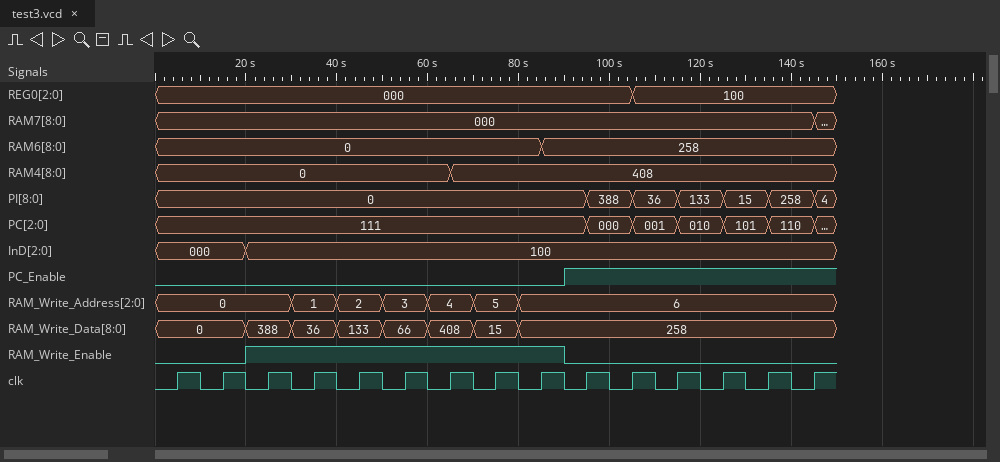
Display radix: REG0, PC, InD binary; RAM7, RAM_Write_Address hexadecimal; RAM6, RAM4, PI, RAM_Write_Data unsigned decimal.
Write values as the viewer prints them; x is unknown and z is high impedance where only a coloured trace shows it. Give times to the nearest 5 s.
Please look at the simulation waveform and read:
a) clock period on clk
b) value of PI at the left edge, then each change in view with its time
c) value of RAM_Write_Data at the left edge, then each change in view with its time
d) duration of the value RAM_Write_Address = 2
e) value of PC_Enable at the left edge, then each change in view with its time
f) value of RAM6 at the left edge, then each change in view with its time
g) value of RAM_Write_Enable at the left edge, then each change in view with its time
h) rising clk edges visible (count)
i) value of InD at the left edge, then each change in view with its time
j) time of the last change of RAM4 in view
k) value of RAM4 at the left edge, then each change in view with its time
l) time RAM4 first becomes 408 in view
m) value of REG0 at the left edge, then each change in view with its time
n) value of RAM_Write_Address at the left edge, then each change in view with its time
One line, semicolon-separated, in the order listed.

10 s; 0, 388 at 95 s, 36 at 105 s, 133 at 115 s, 15 at 125 s, 258 at 135 s, 4 at 145 s; 0, 388 at 20 s, 36 at 30 s, 133 at 40 s, 66 at 50 s, 408 at 60 s, 15 at 70 s, 258 at 80 s; 10 s; 0, 1 at 90 s; 0, 258 at 85 s; 0, 1 at 20 s, 0 at 90 s; 15; 000, 100 at 20 s; 65 s; 0, 408 at 65 s; 65 s; 000, 100 at 105 s; 0, 1 at 30 s, 2 at 40 s, 3 at 50 s, 4 at 60 s, 5 at 70 s, 6 at 80 s
